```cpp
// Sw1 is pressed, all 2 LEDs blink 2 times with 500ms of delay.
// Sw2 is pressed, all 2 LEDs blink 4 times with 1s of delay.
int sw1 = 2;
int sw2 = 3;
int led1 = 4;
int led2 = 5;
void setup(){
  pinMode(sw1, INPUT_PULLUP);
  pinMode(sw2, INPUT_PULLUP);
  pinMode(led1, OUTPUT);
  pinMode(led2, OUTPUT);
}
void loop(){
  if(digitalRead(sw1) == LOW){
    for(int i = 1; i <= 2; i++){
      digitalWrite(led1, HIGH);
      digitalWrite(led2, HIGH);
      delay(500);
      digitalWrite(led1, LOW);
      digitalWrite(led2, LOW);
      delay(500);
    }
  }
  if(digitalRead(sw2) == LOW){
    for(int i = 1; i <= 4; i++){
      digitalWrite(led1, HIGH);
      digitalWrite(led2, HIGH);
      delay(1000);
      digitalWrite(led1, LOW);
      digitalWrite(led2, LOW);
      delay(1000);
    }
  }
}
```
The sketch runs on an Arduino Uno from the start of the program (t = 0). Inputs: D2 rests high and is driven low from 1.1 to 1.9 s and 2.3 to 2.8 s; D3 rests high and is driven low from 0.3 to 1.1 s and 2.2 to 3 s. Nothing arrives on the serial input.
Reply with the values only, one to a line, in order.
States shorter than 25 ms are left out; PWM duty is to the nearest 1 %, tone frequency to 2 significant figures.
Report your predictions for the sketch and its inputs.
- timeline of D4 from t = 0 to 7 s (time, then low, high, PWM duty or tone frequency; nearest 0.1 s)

0 s low; 0.3 s high; 1.3 s low; 2.3 s high; 3.3 s low; 4.3 s high; 5.3 s low; 6.3 s high
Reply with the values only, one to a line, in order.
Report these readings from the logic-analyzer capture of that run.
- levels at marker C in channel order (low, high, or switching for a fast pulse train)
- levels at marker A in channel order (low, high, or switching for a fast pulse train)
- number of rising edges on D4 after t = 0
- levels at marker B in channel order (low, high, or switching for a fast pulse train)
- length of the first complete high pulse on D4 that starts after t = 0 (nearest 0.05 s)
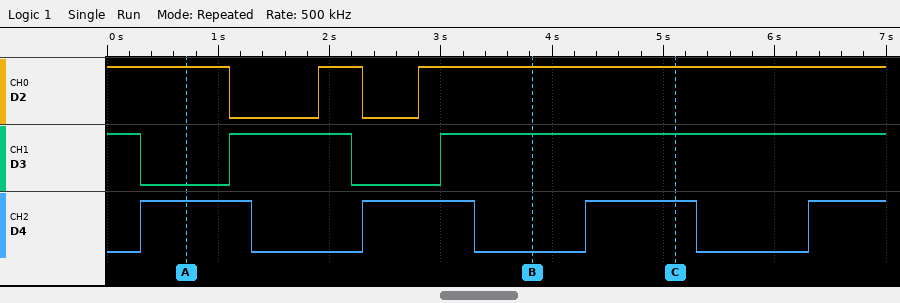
D2 high, D3 high, D4 high
D2 high, D3 low, D4 high
4
D2 high, D3 high, D4 low
1.00 s
